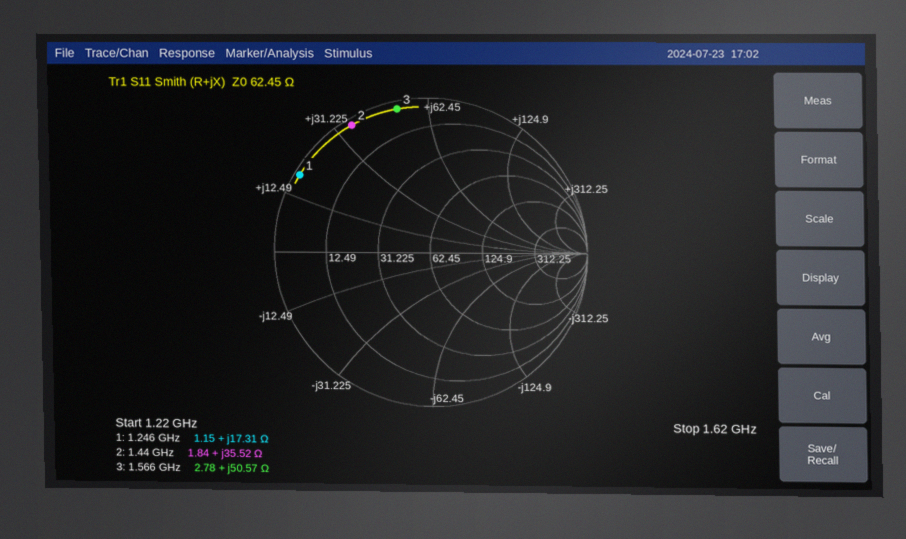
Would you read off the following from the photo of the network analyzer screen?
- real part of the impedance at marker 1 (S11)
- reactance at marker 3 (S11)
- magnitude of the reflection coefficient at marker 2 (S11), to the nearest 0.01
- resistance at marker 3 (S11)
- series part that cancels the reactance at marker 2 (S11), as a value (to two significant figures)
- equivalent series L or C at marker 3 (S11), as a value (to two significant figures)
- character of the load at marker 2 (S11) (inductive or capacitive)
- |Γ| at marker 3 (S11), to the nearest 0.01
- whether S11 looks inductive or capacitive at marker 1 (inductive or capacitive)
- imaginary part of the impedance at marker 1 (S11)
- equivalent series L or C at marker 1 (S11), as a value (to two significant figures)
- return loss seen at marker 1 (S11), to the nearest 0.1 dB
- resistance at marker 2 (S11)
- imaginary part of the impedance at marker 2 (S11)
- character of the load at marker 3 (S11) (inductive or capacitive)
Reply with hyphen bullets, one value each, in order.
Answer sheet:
- 1.15 Ω
- +50.57 Ω
- 0.96
- 2.78 Ω
- 3.1 pF
- 5.1 nH
- inductive
- 0.95
- inductive
- +17.31 Ω
- 2.2 nH
- 0.3 dB
- 1.84 Ω
- +35.52 Ω
- inductive
